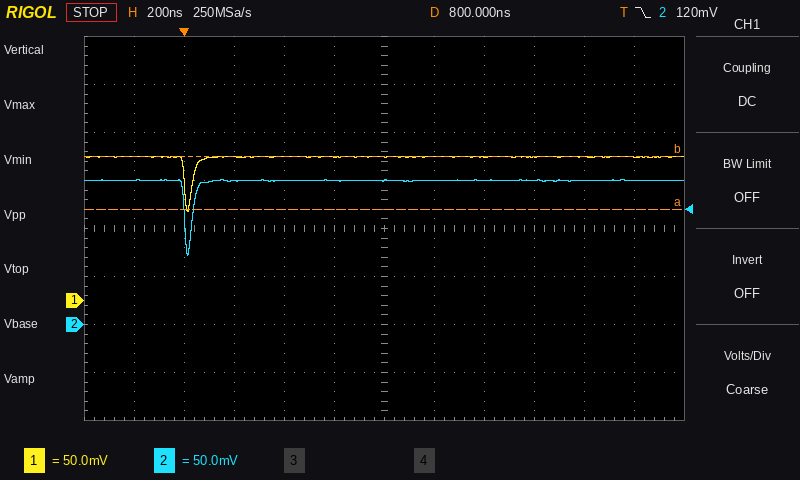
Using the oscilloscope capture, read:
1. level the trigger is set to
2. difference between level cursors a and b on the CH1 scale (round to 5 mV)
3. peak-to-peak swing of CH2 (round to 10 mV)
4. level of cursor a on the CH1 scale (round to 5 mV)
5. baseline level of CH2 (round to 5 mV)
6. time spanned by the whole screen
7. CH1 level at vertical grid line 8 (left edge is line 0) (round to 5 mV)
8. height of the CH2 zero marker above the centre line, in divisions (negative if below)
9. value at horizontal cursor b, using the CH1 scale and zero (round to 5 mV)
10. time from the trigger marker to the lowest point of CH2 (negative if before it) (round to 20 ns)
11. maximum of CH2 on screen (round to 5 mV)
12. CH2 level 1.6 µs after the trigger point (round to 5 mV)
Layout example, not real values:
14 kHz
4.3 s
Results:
120 mV
55 mV
80 mV
95 mV
150 mV
2.4 µs
150 mV
-2.0 div
150 mV
+20 ns
150 mV
150 mV
